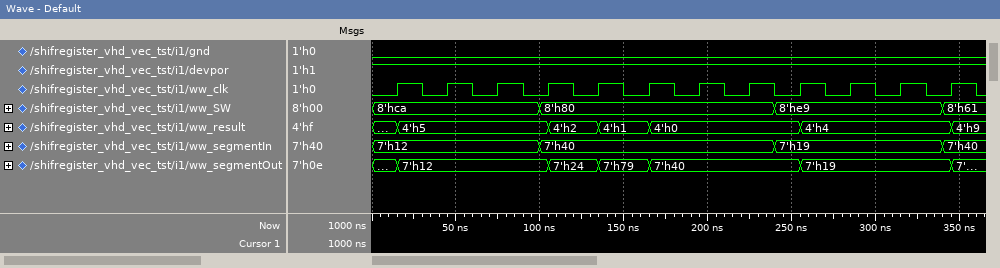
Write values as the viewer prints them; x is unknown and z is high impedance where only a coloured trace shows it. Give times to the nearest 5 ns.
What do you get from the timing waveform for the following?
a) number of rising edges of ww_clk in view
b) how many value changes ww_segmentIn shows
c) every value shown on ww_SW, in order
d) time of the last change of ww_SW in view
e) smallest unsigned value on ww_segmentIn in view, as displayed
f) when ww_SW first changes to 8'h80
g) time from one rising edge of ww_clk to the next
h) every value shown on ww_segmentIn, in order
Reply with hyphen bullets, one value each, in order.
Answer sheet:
- 12
- 3
- 8'hca, 8'h80, 8'he9, 8'h61
- 340 ns
- 7'h12
- 100 ns
- 30 ns
- 7'h12, 7'h40, 7'h19, 7'h40
